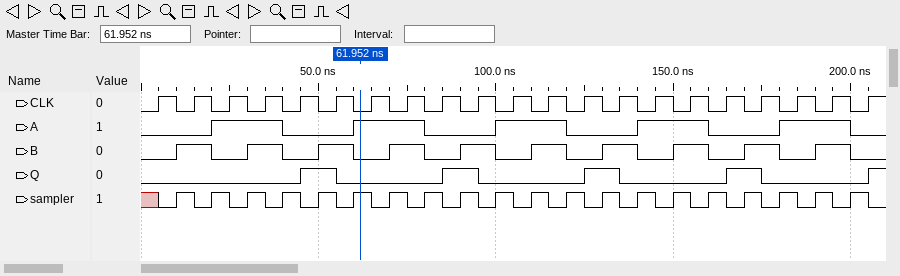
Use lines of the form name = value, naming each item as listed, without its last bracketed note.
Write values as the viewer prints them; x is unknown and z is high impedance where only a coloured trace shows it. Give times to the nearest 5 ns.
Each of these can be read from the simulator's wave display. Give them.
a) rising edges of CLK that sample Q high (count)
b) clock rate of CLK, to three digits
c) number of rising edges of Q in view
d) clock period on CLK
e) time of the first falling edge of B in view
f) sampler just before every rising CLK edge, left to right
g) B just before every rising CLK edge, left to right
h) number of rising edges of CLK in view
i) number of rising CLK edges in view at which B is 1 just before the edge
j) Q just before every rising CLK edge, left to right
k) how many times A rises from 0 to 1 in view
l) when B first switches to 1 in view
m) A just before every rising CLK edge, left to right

rising edges of CLK that sample Q high = 4
clock rate of CLK, to three digits = 100 MHz
number of rising edges of Q in view = 5
clock period on CLK = 10 ns
time of the first falling edge of B in view = 20 ns
sampler just before every rising CLK edge, left to right = x 1 1 1 1 1 1 1 1 1 1 1 1 1 1 1 1 1 1 1 1
B just before every rising CLK edge, left to right = 0 1 0 1 0 1 0 1 0 1 0 1 0 1 0 1 0 1 0 1 0
number of rising edges of CLK in view = 21
number of rising CLK edges in view at which B is 1 just before the edge = 10
Q just before every rising CLK edge, left to right = 0 0 0 0 0 1 0 0 0 1 0 0 0 1 0 0 0 1 0 0 0
how many times A rises from 0 to 1 in view = 5
when B first switches to 1 in view = 10 ns
A just before every rising CLK edge, left to right = 0 0 1 1 0 0 1 1 0 0 1 1 0 0 1 1 0 0 1 1 0
